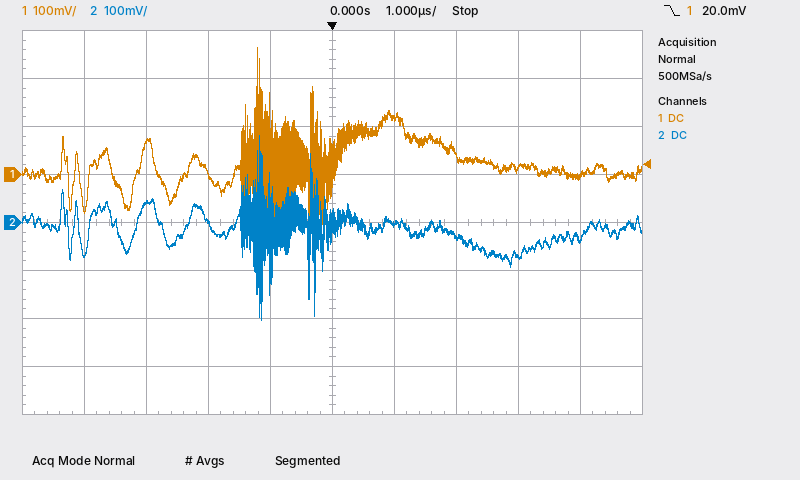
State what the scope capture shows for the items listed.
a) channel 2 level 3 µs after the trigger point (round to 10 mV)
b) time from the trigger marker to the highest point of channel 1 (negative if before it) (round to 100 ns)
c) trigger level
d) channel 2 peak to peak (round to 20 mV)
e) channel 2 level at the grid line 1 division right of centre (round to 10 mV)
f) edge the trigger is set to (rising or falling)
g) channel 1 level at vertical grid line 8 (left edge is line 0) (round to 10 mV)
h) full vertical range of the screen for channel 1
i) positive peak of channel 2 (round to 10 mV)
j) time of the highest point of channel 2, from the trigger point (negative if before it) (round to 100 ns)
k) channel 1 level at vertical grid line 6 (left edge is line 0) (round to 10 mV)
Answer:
-70 mV
-1.2 µs
20.0 mV
380 mV
0 mV
falling
10 mV
800 mV
180 mV
-1.2 µs
120 mV
